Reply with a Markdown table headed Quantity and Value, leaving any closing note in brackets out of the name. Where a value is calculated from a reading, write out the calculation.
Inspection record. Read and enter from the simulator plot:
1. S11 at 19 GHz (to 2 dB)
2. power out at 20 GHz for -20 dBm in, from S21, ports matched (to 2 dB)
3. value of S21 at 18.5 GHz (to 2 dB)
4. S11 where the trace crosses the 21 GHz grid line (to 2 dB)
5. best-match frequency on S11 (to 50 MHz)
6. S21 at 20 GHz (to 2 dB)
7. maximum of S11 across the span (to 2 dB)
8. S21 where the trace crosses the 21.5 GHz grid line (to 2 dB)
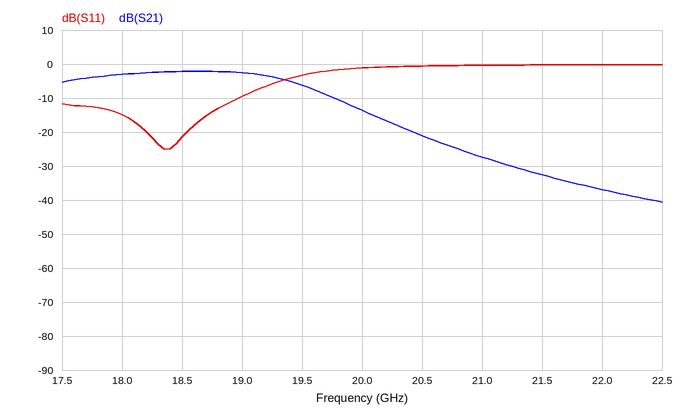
| Quantity | Value |
|---|---|
| S11 at 19 GHz | -10 dB |
| power out at 20 GHz for -20 dBm in, from S21, ports matched | -20 dBm + (-14 dB) = -34 dBm |
| value of S21 at 18.5 GHz | -2 dB |
| S11 where the trace crosses the 21 GHz grid line | 0 dB |
| best-match frequency on S11 | 18.35 GHz |
| S21 at 20 GHz | -14 dB |
| maximum of S11 across the span | 0 dB |
| S21 where the trace crosses the 21.5 GHz grid line | -32 dB |
